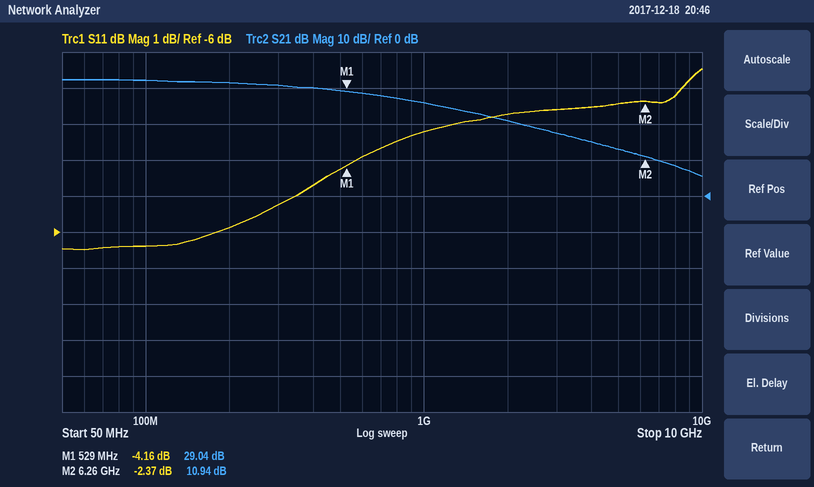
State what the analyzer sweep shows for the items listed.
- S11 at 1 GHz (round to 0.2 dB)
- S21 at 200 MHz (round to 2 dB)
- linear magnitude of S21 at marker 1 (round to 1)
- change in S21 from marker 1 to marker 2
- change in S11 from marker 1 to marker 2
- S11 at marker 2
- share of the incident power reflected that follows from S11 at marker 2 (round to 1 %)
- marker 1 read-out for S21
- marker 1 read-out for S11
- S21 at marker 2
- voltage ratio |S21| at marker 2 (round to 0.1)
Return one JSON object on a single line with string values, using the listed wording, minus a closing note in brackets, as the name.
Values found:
{"S11 at 1 GHz": "-3.2 dB", "S21 at 200 MHz": "32 dB", "linear magnitude of S21 at marker 1": "28", "change in S21 from marker 1 to marker 2": "-18.10 dB", "change in S11 from marker 1 to marker 2": "1.79 dB", "S11 at marker 2": "-2.37 dB", "share of the incident power reflected that follows from S11 at marker 2": "58 %", "marker 1 read-out for S21": "29.04 dB", "marker 1 read-out for S11": "-4.16 dB", "S21 at marker 2": "10.94 dB", "voltage ratio |S21| at marker 2": "3.5"}
